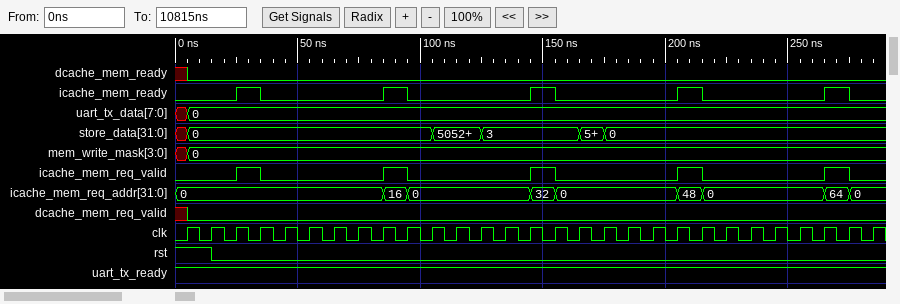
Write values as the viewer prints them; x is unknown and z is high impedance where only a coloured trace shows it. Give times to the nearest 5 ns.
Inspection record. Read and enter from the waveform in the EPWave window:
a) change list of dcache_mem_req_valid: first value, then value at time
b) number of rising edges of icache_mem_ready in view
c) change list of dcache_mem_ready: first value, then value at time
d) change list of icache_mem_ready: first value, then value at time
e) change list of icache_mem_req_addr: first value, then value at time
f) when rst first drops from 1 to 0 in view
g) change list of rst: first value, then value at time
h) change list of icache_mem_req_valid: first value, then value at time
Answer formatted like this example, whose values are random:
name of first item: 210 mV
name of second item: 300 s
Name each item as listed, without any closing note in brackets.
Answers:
change list of dcache_mem_req_valid: first value, then value at time: x, 0 at 5 ns
number of rising edges of icache_mem_ready in view: 5
change list of dcache_mem_ready: first value, then value at time: x, 0 at 5 ns
change list of icache_mem_ready: first value, then value at time: 0, 1 at 25 ns, 0 at 35 ns, 1 at 85 ns, 0 at 95 ns, 1 at 145 ns, 0 at 155 ns, 1 at 205 ns, 0 at 215 ns, 1 at 265 ns, 0 at 275 ns
change list of icache_mem_req_addr: first value, then value at time: 0, 16 at 85 ns, 0 at 95 ns, 32 at 145 ns, 0 at 155 ns, 48 at 205 ns, 0 at 215 ns, 64 at 265 ns, 0 at 275 ns
when rst first drops from 1 to 0 in view: 15 ns
change list of rst: first value, then value at time: 1, 0 at 15 ns
change list of icache_mem_req_valid: first value, then value at time: 0, 1 at 25 ns, 0 at 35 ns, 1 at 85 ns, 0 at 95 ns, 1 at 145 ns, 0 at 155 ns, 1 at 205 ns, 0 at 215 ns, 1 at 265 ns, 0 at 275 ns
